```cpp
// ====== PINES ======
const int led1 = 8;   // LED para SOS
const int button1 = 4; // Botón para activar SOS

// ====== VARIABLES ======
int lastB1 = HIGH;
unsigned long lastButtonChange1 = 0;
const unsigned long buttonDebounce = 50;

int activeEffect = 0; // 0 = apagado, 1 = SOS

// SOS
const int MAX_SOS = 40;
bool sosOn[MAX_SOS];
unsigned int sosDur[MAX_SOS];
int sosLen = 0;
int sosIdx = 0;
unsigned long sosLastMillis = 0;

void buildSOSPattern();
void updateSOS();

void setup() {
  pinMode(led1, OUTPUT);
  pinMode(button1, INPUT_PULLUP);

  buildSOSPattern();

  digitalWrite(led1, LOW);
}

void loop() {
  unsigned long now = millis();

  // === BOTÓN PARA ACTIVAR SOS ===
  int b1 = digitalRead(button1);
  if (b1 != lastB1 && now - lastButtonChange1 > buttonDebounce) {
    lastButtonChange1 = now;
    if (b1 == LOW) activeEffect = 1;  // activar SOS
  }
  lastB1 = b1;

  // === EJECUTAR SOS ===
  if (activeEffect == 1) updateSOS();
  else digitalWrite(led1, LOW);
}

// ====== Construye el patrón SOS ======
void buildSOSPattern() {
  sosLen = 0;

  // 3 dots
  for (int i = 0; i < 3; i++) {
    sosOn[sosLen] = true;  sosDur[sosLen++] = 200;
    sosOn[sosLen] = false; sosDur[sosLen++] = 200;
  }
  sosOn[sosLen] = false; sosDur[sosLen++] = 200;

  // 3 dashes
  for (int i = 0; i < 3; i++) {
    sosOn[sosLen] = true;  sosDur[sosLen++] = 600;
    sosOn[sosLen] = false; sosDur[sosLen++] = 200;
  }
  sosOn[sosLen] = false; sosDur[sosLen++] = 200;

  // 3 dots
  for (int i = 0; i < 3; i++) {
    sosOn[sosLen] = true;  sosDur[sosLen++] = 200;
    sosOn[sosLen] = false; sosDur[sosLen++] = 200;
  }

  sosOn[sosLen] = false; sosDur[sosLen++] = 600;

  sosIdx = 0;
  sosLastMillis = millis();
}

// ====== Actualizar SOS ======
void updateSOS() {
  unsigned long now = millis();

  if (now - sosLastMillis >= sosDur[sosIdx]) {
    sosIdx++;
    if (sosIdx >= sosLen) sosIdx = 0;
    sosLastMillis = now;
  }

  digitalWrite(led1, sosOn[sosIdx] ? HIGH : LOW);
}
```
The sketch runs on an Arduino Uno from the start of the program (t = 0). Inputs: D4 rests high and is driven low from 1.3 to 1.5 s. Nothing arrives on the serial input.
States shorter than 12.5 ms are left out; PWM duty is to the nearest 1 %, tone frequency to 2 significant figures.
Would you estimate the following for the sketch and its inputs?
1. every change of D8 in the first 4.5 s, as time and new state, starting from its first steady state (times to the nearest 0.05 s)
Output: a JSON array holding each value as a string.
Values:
["0 s low; 1.5 s high; 1.7 s low; 1.9 s high; 2.1 s low; 2.5 s high; 3.1 s low; 3.3 s high; 3.9 s low; 4.1 s high"]
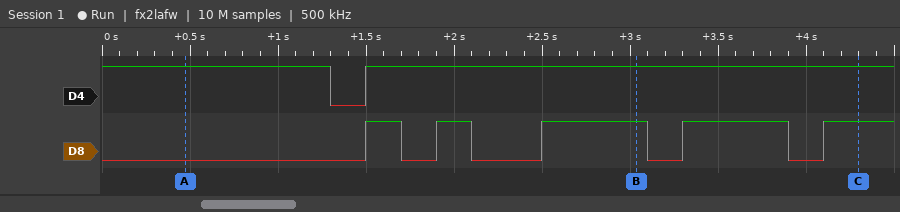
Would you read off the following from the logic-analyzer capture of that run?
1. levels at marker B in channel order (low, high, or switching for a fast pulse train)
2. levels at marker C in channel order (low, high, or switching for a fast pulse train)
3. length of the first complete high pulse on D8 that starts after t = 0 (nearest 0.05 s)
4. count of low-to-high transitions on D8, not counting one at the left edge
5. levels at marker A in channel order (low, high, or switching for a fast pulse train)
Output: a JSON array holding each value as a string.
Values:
["D4 high, D8 high", "D4 high, D8 high", "0.20 s", "5", "D4 high, D8 low"]
